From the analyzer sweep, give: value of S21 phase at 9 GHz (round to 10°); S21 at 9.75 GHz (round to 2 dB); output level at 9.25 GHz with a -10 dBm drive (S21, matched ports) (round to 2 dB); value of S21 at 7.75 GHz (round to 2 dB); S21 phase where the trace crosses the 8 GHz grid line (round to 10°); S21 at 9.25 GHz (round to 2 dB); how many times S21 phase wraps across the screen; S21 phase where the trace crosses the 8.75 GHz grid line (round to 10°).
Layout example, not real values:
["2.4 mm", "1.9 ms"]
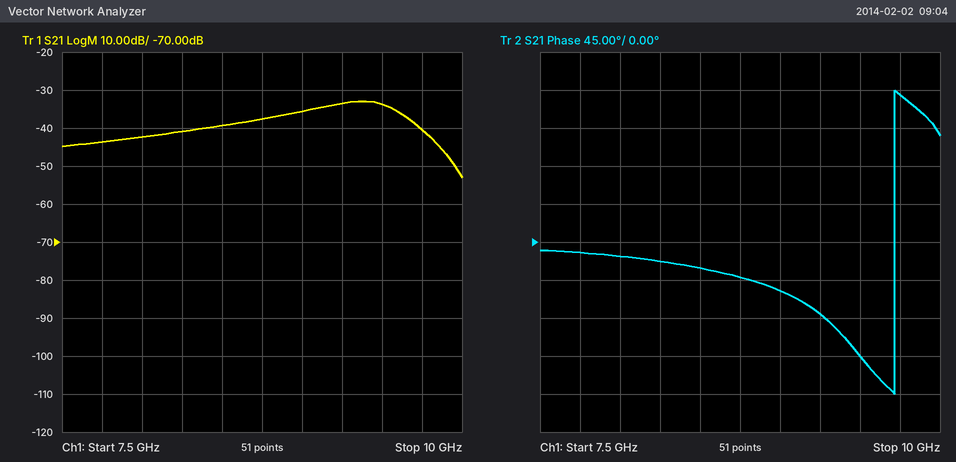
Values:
["-60°", "-40 dB", "-44 dBm", "-44 dB", "-20°", "-34 dB", "1", "-40°"]
